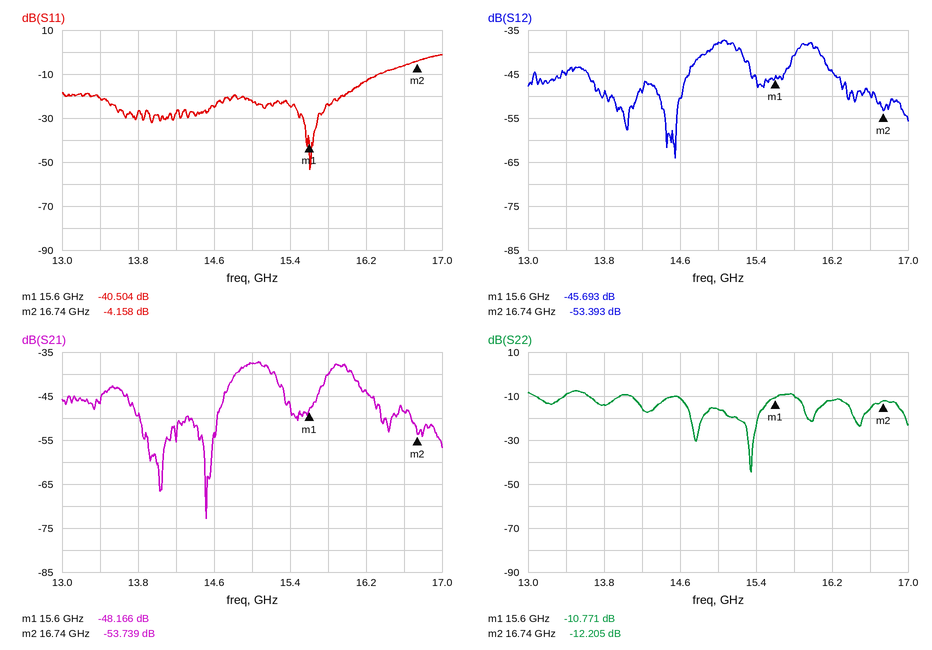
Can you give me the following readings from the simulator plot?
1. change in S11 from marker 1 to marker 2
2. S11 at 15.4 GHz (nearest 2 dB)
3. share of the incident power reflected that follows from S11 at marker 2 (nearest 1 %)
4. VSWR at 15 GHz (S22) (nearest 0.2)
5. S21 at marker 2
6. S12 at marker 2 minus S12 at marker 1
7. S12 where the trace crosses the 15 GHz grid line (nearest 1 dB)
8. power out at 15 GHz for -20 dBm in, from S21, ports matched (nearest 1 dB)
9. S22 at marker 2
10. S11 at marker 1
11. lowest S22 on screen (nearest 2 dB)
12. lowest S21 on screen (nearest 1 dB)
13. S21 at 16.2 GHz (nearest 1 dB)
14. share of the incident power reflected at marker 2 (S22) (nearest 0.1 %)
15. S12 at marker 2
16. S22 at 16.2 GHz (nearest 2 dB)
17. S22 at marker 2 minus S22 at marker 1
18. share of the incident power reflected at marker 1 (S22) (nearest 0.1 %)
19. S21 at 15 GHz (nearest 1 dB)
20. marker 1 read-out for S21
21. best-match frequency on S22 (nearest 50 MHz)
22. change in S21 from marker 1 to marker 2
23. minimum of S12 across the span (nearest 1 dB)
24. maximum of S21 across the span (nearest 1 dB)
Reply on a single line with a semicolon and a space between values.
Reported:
36.346 dB; -24 dB; 38 %; 1.4; -53.739 dB; -7.700 dB; -38 dB; -58 dBm; -12.205 dB; -40.504 dB; -44 dB; -73 dB; -44 dB; 6.0 %; -53.393 dB; -12 dB; -1.434 dB; 8.4 %; -38 dB; -48.166 dB; 15.35 GHz; -5.573 dB; -64 dB; -37 dB
